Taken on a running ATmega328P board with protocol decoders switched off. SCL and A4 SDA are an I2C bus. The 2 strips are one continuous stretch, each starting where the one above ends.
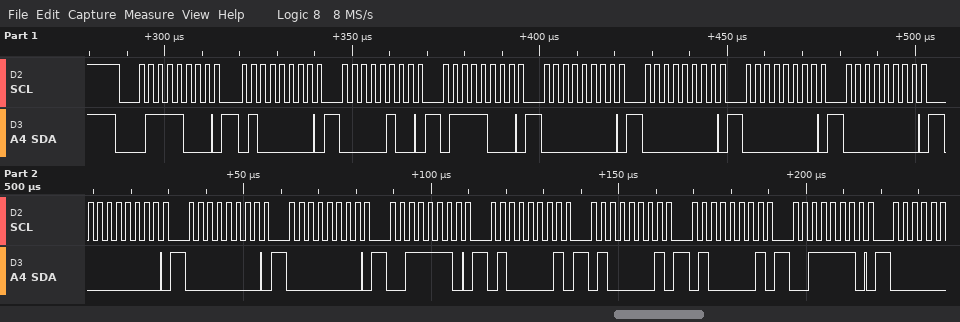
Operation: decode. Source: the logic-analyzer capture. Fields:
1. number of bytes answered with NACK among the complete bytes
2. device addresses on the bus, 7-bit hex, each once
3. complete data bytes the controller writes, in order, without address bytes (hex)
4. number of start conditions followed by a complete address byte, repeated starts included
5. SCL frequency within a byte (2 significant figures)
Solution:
0
0x3C
40 04 78 00 00 00 00 00 00 00 3E 41 41 41 3E
1
400 kHz
